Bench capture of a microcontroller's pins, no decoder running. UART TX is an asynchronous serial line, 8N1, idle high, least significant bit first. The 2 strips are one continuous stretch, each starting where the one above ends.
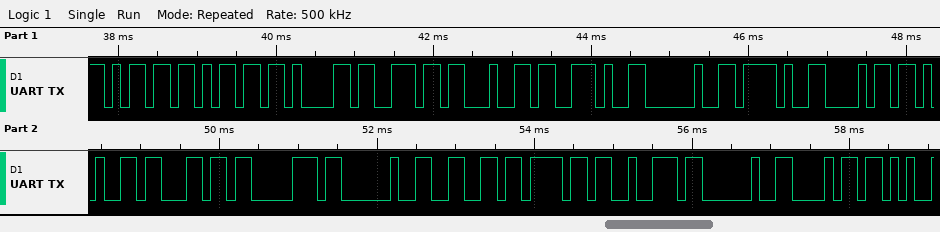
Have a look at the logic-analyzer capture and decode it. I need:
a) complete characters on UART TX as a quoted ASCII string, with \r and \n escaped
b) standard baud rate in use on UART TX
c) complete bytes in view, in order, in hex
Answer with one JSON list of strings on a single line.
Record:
["\"mmand. /help for h\"", "9600 baud", "6D 6D 61 6E 64 2E 20 2F 68 65 6C 70 20 66 6F 72 20 68"]
